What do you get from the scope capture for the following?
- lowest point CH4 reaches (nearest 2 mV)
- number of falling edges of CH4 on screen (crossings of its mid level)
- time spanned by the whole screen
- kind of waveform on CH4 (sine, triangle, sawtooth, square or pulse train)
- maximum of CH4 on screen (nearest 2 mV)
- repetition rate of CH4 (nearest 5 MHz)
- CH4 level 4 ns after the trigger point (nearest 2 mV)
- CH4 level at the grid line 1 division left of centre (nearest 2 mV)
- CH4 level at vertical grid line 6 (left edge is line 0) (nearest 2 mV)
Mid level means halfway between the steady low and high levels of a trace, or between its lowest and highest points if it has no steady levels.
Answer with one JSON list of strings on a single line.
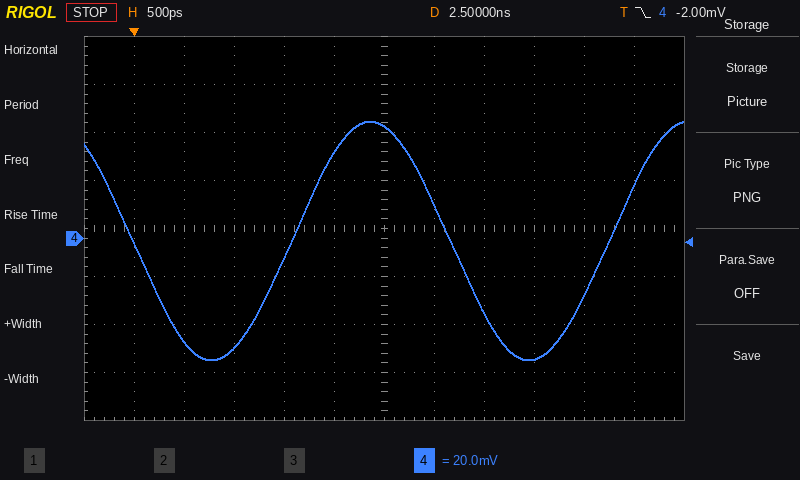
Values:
["-50 mV", "2", "6 ns", "sine", "48 mV", "315 MHz", "-50 mV", "36 mV", "46 mV"]
